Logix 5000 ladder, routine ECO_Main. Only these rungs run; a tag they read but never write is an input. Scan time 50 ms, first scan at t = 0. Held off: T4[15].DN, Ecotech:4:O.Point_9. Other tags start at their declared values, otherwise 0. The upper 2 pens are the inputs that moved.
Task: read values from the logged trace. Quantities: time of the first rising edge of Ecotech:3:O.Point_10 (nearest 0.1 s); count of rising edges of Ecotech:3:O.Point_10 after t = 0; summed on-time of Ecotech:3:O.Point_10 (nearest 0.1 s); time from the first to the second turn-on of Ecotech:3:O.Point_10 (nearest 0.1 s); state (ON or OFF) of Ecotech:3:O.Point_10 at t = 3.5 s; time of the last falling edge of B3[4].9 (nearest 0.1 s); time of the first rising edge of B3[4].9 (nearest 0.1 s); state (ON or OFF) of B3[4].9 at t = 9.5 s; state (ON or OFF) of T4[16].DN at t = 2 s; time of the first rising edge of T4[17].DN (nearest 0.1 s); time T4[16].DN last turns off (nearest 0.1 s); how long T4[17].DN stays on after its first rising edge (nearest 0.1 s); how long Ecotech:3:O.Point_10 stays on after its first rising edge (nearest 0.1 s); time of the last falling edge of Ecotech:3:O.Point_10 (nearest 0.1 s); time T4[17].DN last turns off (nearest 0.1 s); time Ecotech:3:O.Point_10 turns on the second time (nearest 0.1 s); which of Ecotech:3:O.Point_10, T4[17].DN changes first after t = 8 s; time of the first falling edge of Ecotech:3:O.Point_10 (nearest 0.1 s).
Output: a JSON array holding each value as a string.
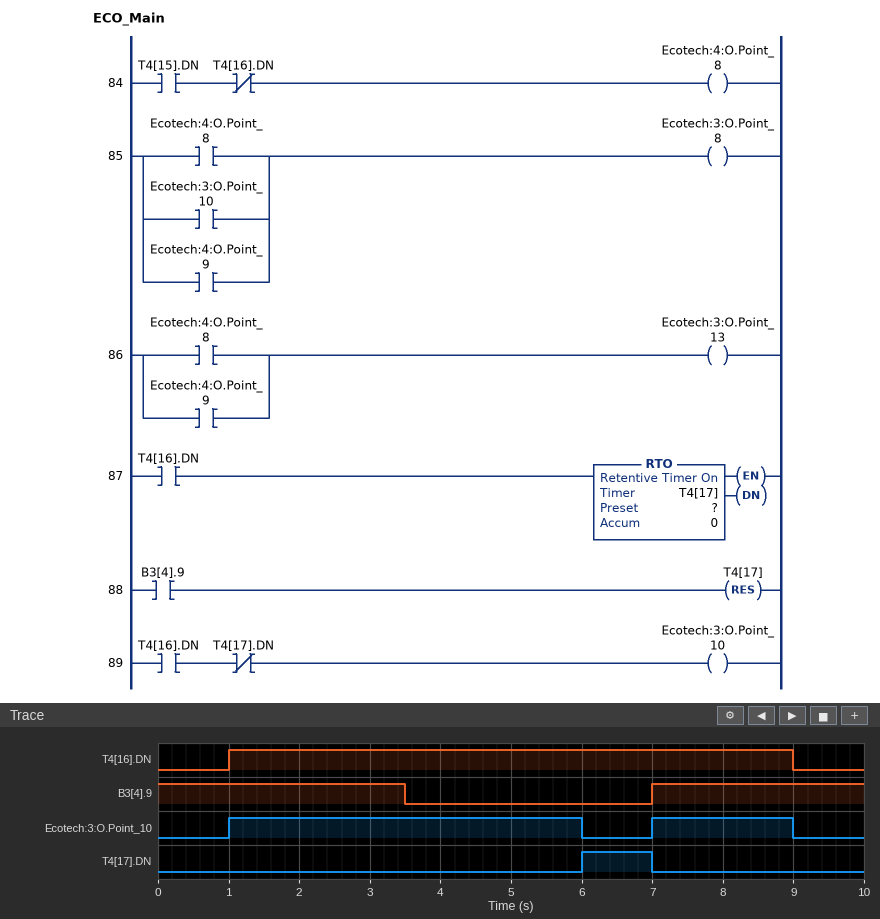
["1.0 s", "2", "7.0 s", "6.0 s", "ON", "3.5 s", "7.0 s", "ON", "ON", "6.0 s", "9.0 s", "1.0 s", "5.0 s", "9.0 s", "7.0 s", "7.0 s", "Ecotech:3:O.Point_10", "6.0 s"]
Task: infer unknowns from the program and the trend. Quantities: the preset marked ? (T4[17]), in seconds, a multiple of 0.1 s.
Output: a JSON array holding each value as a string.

["2.5 s"]
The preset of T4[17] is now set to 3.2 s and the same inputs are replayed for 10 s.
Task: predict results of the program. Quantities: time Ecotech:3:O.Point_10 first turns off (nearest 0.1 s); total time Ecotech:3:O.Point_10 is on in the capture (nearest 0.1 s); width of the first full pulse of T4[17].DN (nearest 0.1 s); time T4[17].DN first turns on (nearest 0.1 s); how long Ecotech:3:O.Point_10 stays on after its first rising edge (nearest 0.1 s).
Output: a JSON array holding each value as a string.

["6.7 s", "7.7 s", "0.3 s", "6.7 s", "5.7 s"]
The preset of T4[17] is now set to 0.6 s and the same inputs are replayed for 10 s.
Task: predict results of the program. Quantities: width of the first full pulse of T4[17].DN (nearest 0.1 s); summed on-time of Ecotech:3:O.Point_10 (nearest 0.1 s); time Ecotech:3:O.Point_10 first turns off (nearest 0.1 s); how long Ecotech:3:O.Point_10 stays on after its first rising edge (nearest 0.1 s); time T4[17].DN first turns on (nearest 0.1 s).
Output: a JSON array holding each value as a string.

["2.9 s", "5.1 s", "4.1 s", "3.1 s", "4.1 s"]
